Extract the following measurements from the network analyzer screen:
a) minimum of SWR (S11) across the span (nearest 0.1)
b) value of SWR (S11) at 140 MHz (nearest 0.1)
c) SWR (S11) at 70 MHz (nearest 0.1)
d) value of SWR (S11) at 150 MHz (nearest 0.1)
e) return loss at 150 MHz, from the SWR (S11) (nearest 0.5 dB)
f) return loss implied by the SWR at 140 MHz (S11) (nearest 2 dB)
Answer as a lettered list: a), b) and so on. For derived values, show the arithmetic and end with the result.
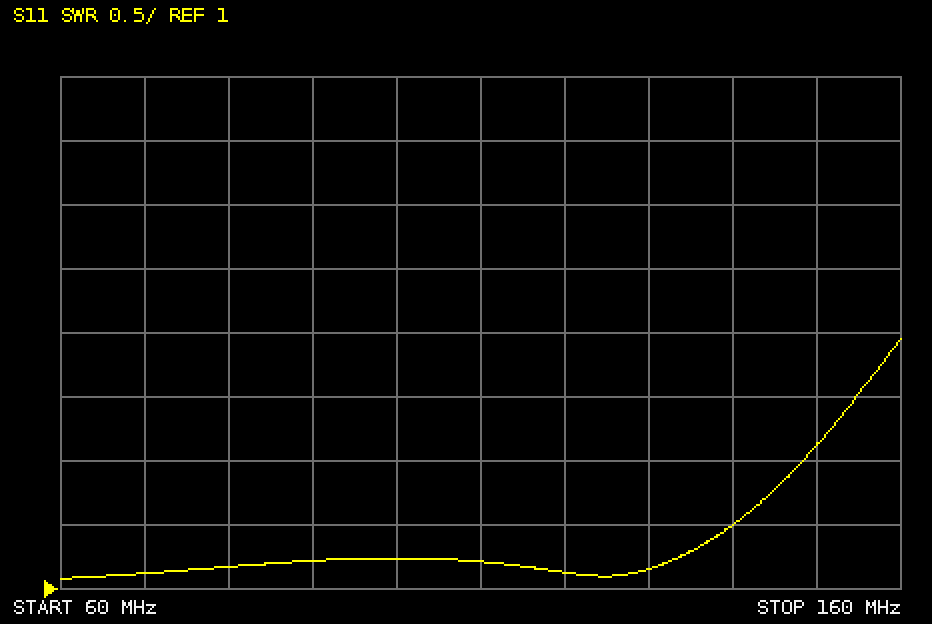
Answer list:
a) 1.1
b) 1.5
c) 1.1
d) 2.1
e) −20 log10((2.1 − 1)/(2.1 + 1)) ≈ 9.0 dB
f) −20 log10((1.5 − 1)/(1.5 + 1)) ≈ 14 dB
